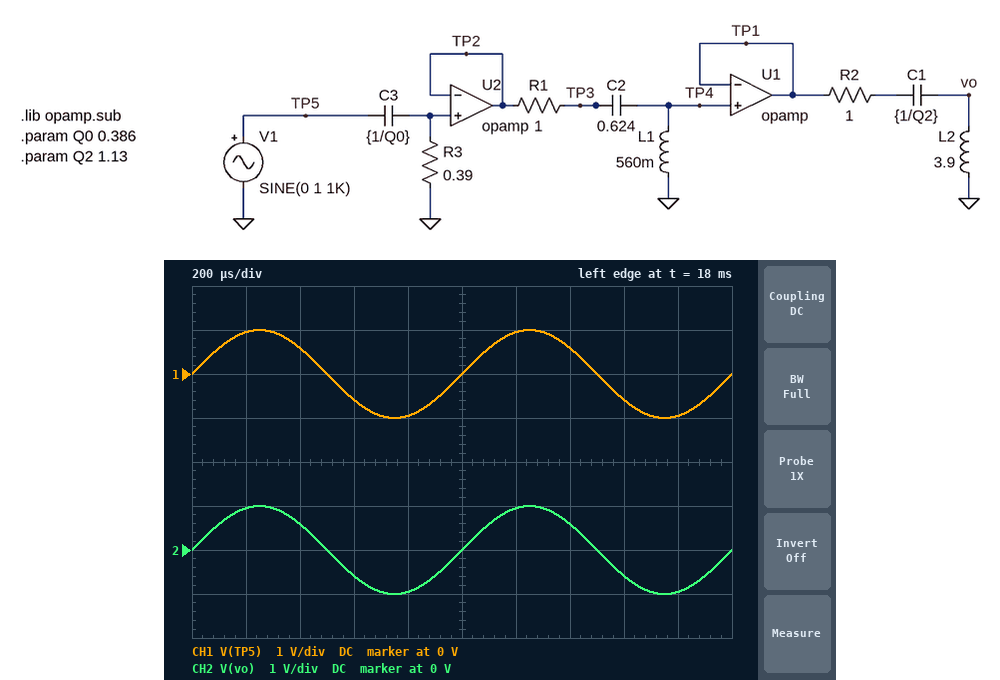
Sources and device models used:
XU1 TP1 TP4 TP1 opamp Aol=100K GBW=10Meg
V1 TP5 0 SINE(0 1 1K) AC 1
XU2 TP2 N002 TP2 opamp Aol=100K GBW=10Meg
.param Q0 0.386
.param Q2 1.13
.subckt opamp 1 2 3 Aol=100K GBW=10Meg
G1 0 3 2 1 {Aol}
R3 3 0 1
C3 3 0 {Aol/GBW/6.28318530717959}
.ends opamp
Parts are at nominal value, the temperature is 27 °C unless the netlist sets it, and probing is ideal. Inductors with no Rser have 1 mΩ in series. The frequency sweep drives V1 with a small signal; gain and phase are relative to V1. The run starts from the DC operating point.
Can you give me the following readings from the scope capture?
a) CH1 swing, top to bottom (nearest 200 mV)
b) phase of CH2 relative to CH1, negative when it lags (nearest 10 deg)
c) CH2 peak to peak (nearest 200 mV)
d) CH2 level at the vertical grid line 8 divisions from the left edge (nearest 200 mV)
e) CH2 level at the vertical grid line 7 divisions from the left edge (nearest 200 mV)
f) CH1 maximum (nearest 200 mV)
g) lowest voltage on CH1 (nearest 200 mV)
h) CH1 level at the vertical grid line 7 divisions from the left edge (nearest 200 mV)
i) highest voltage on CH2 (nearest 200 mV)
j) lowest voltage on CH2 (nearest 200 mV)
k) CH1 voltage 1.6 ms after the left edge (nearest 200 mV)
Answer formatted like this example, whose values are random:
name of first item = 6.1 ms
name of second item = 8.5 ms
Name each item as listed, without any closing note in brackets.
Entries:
CH1 swing, top to bottom = 2.0 V
phase of CH2 relative to CH1, negative when it lags = 0 deg
CH2 peak to peak = 2.0 V
CH2 level at the vertical grid line 8 divisions from the left edge = -600 mV
CH2 level at the vertical grid line 7 divisions from the left edge = 600 mV
CH1 maximum = 1.0 V
lowest voltage on CH1 = -1.0 V
CH1 level at the vertical grid line 7 divisions from the left edge = 600 mV
highest voltage on CH2 = 1.0 V
lowest voltage on CH2 = -1.0 V
CH1 voltage 1.6 ms after the left edge = -600 mV
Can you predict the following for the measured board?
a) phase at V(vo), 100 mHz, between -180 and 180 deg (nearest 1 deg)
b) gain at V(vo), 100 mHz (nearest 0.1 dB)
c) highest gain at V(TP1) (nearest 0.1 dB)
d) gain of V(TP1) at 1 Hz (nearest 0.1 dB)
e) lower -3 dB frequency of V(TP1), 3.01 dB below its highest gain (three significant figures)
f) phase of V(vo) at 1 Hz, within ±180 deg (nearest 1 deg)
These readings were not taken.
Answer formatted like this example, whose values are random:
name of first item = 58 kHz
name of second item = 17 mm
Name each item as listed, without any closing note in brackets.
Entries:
phase at V(vo), 100 mHz, between -180 and 180 deg = -90 deg
gain at V(vo), 100 mHz = -15.9 dB
highest gain at V(TP1) = 0.4 dB
gain of V(TP1) at 1 Hz = 0.2 dB
lower -3 dB frequency of V(TP1), 3.01 dB below its highest gain = 251 mHz
phase of V(vo) at 1 Hz, within ±180 deg = 28 deg
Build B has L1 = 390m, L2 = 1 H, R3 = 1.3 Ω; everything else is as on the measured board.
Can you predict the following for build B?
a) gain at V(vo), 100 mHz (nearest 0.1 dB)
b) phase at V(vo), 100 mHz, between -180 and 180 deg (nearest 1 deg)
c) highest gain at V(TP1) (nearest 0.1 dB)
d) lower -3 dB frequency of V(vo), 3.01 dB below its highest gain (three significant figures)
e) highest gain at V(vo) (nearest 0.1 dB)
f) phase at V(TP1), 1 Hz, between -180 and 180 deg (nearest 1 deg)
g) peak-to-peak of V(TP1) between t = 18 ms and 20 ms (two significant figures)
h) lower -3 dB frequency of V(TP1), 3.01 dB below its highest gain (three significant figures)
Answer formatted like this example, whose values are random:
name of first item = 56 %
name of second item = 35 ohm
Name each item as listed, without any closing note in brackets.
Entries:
gain at V(vo), 100 mHz = -28.9 dB
phase at V(vo), 100 mHz, between -180 and 180 deg = -39 deg
highest gain at V(TP1) = 0.2 dB
lower -3 dB frequency of V(vo), 3.01 dB below its highest gain = 272 mHz
highest gain at V(vo) = 0.5 dB
phase at V(TP1), 1 Hz, between -180 and 180 deg = 27 deg
peak-to-peak of V(TP1) between t = 18 ms and 20 ms = 2.0 V
lower -3 dB frequency of V(TP1), 3.01 dB below its highest gain = 300 mHz
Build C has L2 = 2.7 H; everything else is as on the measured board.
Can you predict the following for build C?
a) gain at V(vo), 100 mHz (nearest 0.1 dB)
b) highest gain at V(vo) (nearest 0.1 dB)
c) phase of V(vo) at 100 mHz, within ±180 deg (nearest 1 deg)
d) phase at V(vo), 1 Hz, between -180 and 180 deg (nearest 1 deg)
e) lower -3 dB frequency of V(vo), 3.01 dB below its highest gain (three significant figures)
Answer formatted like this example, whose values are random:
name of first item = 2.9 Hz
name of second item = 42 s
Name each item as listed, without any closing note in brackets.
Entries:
gain at V(vo), 100 mHz = -17.6 dB
highest gain at V(vo) = 0.8 dB
phase of V(vo) at 100 mHz, within ±180 deg = -51 deg
phase at V(vo), 1 Hz, between -180 and 180 deg = 29 deg
lower -3 dB frequency of V(vo), 3.01 dB below its highest gain = 233 mHz
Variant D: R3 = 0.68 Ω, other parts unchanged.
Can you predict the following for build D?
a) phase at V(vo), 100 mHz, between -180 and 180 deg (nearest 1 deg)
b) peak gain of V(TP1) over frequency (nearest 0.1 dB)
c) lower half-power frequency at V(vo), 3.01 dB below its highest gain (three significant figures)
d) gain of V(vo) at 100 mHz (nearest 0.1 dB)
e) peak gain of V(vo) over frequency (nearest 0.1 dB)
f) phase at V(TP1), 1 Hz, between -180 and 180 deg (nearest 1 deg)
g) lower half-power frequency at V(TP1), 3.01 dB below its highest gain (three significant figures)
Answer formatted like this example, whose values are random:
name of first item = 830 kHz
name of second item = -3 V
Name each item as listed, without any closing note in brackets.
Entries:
phase at V(vo), 100 mHz, between -180 and 180 deg = -106 deg
peak gain of V(TP1) over frequency = 0.7 dB
lower half-power frequency at V(vo), 3.01 dB below its highest gain = 226 mHz
gain of V(vo) at 100 mHz = -13.1 dB
peak gain of V(vo) over frequency = 1.1 dB
phase at V(TP1), 1 Hz, between -180 and 180 deg = 22 deg
lower half-power frequency at V(TP1), 3.01 dB below its highest gain = 240 mHz
